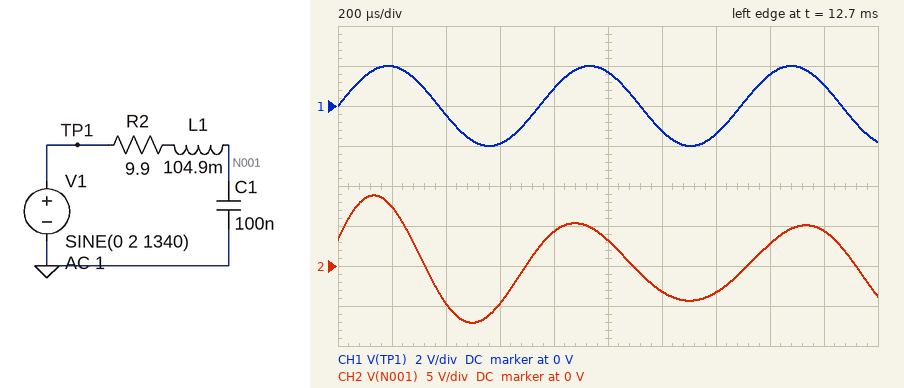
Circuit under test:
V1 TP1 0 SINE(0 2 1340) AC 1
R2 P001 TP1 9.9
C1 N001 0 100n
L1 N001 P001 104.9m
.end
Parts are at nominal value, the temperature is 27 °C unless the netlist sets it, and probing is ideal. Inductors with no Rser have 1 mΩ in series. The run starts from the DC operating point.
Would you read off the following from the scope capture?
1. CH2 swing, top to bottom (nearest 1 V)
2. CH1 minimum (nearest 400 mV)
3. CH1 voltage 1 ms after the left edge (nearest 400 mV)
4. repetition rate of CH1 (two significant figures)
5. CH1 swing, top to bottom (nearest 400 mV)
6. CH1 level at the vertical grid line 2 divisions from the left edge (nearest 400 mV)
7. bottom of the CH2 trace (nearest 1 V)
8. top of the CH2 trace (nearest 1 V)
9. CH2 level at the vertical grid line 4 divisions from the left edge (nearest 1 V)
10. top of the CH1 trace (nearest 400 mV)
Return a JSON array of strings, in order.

["16 V", "-2.0 V", "1.6 V", "1.3 kHz", "4.0 V", "-400 mV", "-7 V", "9 V", "4 V", "2.0 V"]
